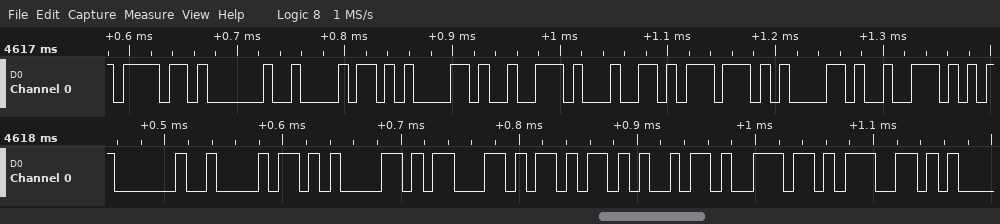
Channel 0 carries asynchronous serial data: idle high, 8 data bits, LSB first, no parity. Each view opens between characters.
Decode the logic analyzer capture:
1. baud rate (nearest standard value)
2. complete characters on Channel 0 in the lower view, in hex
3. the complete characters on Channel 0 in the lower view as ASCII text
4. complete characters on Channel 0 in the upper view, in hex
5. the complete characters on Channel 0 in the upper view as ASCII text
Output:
115200 baud
20, 68, 61, 63, 6B, 69, 6E, 67
" hacking"
6F, 20, 68, 61, 72, 64, 77, 61, 72
"o hardwar"
